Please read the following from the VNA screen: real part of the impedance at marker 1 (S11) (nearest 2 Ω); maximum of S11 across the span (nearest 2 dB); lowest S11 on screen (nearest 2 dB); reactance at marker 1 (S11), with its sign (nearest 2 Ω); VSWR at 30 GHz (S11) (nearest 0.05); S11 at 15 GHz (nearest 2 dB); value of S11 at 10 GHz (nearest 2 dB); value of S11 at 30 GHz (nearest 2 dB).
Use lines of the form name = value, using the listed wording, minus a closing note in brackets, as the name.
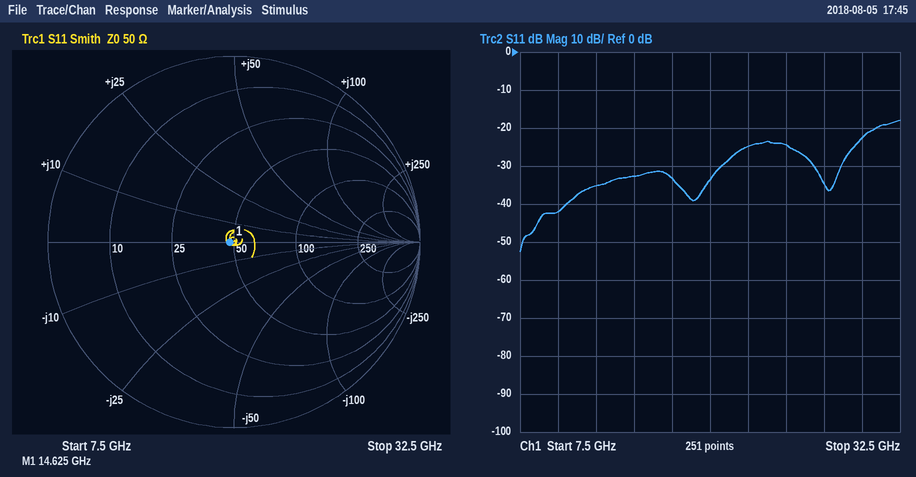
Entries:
real part of the impedance at marker 1 (S11) = 48 Ω
maximum of S11 across the span = -18 dB
lowest S11 on screen = -52 dB
reactance at marker 1 (S11), with its sign = 0 Ω
VSWR at 30 GHz (S11) = 1.15
S11 at 15 GHz = -32 dB
value of S11 at 10 GHz = -42 dB
value of S11 at 30 GHz = -22 dB
